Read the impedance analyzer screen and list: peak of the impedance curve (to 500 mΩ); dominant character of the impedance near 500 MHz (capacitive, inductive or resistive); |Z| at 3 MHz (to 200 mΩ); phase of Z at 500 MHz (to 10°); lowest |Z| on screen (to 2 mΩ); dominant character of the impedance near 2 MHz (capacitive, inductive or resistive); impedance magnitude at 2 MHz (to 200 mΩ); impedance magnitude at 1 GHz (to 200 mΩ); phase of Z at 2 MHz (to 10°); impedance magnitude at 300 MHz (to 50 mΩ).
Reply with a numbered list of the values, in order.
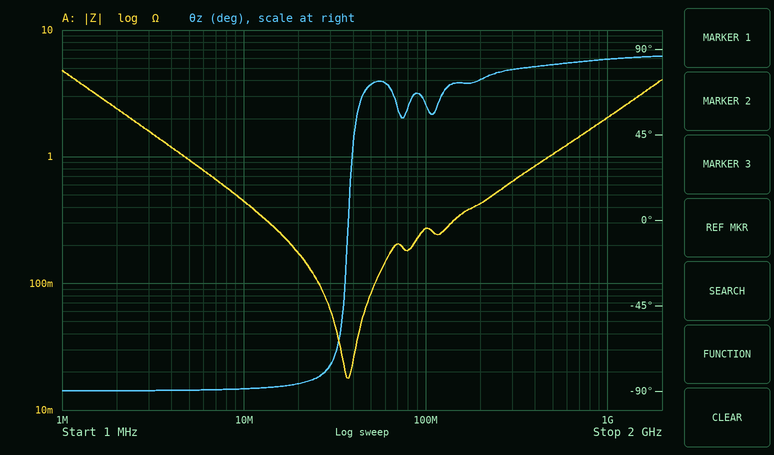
1. 5.0 Ω
2. inductive
3. 1.6 Ω
4. 80°
5. 18 mΩ
6. capacitive
7. 2.4 Ω
8. 2.0 Ω
9. -90°
10. 650 mΩ
